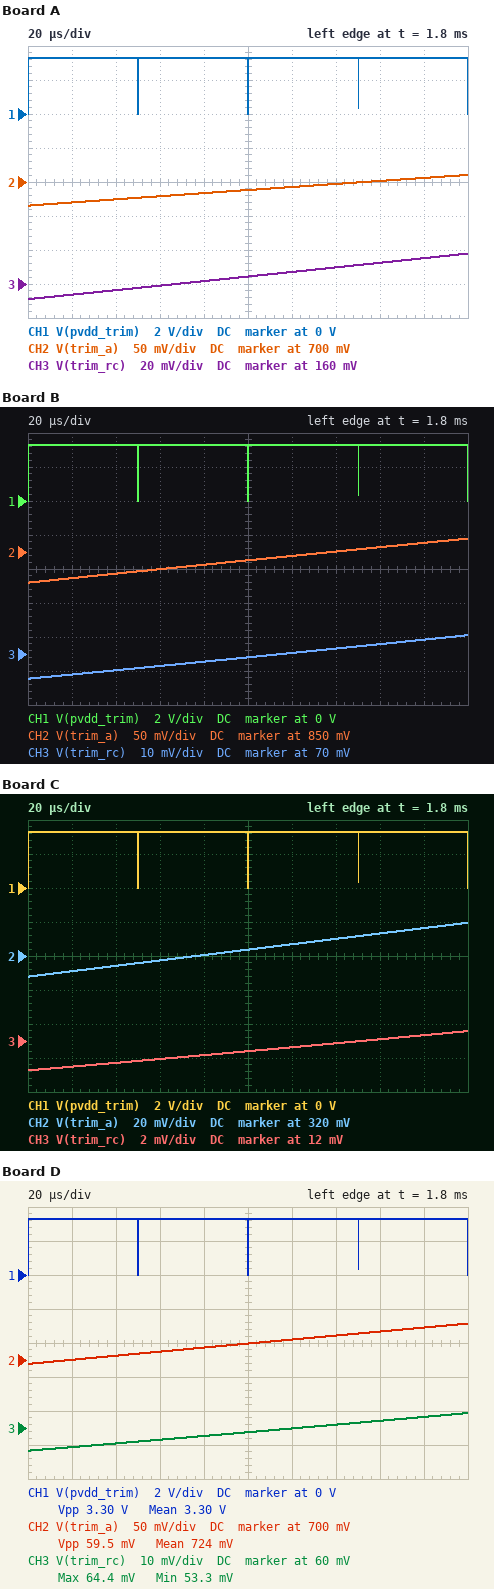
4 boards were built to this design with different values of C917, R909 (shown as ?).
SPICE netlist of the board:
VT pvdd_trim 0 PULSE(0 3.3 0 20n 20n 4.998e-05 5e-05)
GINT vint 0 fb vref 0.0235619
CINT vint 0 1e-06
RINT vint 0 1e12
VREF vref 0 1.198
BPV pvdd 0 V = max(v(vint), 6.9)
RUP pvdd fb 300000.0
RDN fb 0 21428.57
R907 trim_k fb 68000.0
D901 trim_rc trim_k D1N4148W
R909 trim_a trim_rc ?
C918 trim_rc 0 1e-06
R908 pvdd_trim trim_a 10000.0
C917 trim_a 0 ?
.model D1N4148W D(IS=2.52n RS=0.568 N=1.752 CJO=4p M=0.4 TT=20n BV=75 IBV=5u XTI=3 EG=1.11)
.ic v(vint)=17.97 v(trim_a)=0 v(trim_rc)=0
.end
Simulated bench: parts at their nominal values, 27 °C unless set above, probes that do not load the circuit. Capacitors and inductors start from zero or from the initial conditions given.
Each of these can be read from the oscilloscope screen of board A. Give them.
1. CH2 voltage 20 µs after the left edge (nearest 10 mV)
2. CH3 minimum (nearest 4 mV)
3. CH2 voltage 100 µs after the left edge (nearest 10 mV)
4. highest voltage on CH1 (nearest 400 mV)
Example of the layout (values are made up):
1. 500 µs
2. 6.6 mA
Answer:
1. 670 mV
2. 152 mV
3. 690 mV
4. 3.2 V
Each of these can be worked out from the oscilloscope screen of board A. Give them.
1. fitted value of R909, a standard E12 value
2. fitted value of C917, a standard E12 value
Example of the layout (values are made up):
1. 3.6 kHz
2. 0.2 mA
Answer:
1. 3.9 kΩ
2. 560 nF
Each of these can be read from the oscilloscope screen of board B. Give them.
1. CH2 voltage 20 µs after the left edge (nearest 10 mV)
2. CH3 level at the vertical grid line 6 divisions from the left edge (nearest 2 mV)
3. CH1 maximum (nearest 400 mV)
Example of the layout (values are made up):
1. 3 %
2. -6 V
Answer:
1. 810 mV
2. 70 mV
3. 3.2 V
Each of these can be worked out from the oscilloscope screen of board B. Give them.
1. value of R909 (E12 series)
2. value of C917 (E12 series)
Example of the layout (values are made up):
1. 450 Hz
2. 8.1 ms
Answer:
1. 12 kΩ
2. 560 nF
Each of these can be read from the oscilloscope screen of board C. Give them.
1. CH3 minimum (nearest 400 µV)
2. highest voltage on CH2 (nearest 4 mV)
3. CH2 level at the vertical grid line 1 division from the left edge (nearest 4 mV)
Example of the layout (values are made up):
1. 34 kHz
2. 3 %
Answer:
1. 10.4 mV
2. 340 mV
3. 312 mV
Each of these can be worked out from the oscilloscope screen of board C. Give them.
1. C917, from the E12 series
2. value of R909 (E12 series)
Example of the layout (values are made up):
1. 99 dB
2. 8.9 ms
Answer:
1. 1.8 µF
2. 27 kΩ
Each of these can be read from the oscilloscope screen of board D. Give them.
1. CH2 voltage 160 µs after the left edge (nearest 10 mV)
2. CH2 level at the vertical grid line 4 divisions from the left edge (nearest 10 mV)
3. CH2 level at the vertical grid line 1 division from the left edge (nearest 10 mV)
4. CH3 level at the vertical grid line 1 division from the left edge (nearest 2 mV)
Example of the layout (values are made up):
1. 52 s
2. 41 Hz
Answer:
1. 740 mV
2. 720 mV
3. 700 mV
4. 54 mV
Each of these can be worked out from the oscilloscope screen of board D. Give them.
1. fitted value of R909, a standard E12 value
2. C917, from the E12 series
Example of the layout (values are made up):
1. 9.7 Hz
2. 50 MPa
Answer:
1. 12 kΩ
2. 680 nF
